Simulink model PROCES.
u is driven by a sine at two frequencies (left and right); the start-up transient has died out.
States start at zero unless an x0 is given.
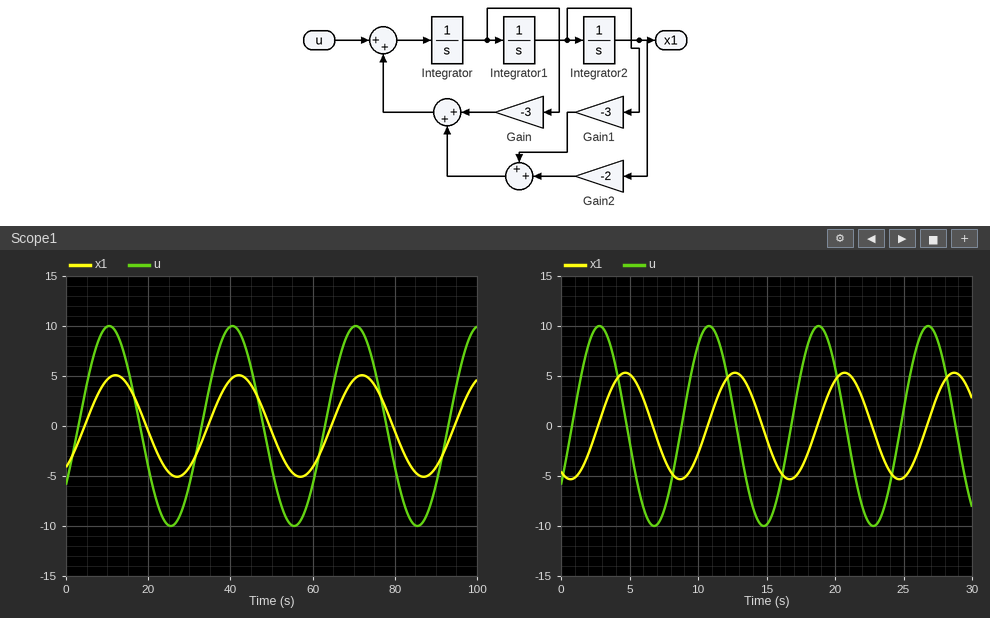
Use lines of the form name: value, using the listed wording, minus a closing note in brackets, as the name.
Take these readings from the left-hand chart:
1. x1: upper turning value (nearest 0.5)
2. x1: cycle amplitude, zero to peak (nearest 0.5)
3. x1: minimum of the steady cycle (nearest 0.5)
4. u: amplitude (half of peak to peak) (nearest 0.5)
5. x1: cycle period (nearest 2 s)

x1: upper turning value: 5.0
x1: cycle amplitude, zero to peak: 5.0
x1: minimum of the steady cycle: -5.0
u: amplitude (half of peak to peak): 10.0
x1: cycle period: 30 s
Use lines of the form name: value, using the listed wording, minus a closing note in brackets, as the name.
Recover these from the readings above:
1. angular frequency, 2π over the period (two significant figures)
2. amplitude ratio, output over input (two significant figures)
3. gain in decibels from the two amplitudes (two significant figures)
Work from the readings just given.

angular frequency, 2π over the period: 0.21 rad/s
amplitude ratio, output over input: 0.50
gain in decibels from the two amplitudes: -6.0 dB
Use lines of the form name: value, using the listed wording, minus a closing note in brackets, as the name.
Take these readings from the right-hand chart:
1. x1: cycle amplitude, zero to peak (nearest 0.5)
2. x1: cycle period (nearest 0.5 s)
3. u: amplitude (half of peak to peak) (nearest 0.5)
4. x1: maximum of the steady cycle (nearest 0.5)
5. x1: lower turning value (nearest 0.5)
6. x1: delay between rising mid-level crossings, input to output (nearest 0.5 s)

x1: cycle amplitude, zero to peak: 5.5
x1: cycle period: 8.0 s
u: amplitude (half of peak to peak): 10.0
x1: maximum of the steady cycle: 5.5
x1: lower turning value: -5.5
x1: delay between rising mid-level crossings, input to output: 2.0 s
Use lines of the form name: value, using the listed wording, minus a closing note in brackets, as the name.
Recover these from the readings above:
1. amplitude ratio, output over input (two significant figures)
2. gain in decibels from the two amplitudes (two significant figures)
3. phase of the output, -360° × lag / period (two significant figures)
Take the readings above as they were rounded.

amplitude ratio, output over input: 0.55
gain in decibels from the two amplitudes: -5.2 dB
phase of the output, -360° × lag / period: -90°
